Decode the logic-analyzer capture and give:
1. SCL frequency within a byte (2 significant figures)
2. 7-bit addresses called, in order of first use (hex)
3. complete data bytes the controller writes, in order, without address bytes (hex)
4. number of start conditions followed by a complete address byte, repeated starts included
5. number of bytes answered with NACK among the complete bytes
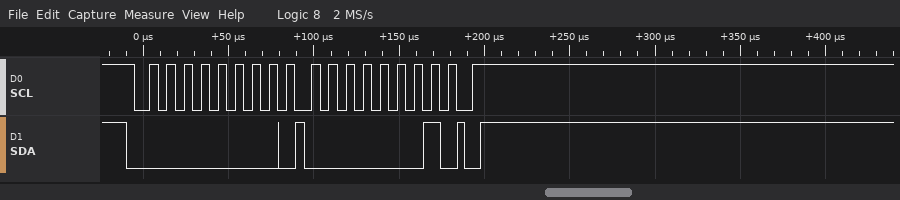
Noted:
100 kHz
0x00
01
1
0
